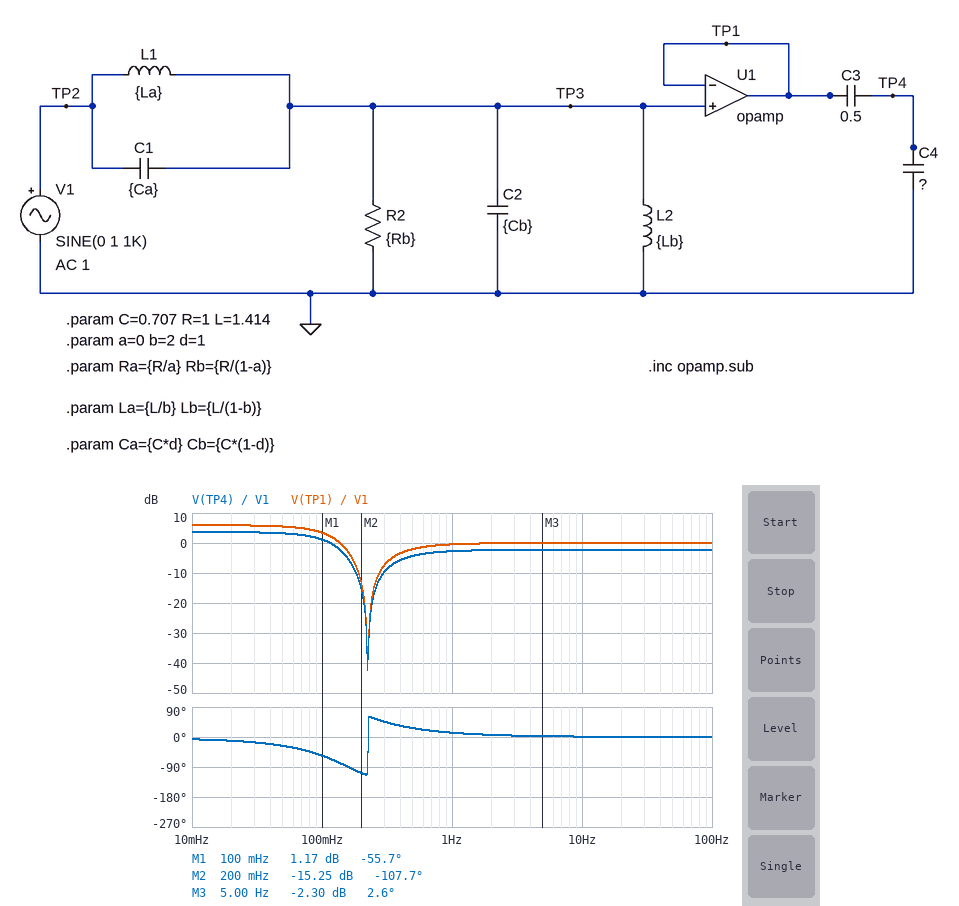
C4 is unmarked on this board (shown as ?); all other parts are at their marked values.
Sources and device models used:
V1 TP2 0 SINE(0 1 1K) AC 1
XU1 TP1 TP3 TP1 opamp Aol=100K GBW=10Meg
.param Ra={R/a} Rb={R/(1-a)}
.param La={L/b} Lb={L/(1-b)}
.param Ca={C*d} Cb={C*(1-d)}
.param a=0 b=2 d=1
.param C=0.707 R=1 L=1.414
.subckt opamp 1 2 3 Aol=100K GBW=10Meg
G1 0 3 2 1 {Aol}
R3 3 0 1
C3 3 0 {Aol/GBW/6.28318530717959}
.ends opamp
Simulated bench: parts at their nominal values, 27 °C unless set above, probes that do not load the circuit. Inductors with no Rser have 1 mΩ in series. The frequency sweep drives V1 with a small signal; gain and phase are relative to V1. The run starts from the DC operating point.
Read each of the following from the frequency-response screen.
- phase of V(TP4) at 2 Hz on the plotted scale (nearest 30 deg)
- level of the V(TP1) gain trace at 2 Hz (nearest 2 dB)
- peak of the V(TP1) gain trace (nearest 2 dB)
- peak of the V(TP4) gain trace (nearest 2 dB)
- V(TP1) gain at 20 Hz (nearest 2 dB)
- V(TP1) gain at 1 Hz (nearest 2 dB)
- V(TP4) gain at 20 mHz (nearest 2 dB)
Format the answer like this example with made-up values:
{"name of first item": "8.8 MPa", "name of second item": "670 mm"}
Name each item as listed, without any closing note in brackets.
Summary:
{"phase of V(TP4) at 2 Hz on the plotted scale": "0 deg", "level of the V(TP1) gain trace at 2 Hz": "0 dB", "peak of the V(TP1) gain trace": "6 dB", "peak of the V(TP4) gain trace": "4 dB", "V(TP1) gain at 20 Hz": "0 dB", "V(TP1) gain at 1 Hz": "0 dB", "V(TP4) gain at 20 mHz": "4 dB"}
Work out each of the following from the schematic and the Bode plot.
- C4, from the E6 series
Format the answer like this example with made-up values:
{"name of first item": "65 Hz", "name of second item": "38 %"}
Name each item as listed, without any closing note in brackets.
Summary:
{"C4, from the E6 series": "150 mF"}
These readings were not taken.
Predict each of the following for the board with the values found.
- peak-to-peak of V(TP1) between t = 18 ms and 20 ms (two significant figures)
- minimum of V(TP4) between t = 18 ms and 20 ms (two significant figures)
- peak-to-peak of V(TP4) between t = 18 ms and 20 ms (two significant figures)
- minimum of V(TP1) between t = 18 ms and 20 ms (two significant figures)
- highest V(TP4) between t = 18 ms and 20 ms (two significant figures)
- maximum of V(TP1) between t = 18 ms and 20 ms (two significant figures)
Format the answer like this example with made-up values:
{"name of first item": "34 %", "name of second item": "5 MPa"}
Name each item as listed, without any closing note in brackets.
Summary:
{"peak-to-peak of V(TP1) between t = 18 ms and 20 ms": "2.0 V", "minimum of V(TP4) between t = 18 ms and 20 ms": "-770 mV", "peak-to-peak of V(TP4) between t = 18 ms and 20 ms": "1.5 V", "minimum of V(TP1) between t = 18 ms and 20 ms": "-1.0 V", "highest V(TP4) between t = 18 ms and 20 ms": "770 mV", "maximum of V(TP1) between t = 18 ms and 20 ms": "1.0 V"}
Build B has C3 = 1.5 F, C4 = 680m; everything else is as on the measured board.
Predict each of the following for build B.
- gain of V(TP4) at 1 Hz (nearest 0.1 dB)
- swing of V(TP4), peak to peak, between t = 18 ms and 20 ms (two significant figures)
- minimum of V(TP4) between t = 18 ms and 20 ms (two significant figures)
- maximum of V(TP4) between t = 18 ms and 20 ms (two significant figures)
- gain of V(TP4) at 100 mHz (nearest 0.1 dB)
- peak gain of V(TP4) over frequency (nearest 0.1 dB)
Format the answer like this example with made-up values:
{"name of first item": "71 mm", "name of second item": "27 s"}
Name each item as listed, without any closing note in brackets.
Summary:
{"gain of V(TP4) at 1 Hz": "-3.7 dB", "swing of V(TP4), peak to peak, between t = 18 ms and 20 ms": "1.4 V", "minimum of V(TP4) between t = 18 ms and 20 ms": "-690 mV", "maximum of V(TP4) between t = 18 ms and 20 ms": "690 mV", "gain of V(TP4) at 100 mHz": "0.2 dB", "peak gain of V(TP4) over frequency": "2.7 dB"}
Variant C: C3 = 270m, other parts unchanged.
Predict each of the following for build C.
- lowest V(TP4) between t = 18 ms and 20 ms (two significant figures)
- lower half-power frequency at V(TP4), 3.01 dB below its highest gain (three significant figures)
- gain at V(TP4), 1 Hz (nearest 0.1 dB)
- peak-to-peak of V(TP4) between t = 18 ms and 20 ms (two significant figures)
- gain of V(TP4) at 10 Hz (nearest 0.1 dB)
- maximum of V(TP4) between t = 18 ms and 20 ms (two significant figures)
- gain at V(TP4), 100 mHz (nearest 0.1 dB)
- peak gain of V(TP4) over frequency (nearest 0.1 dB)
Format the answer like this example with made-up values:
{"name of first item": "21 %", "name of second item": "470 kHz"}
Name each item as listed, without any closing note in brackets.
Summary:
{"lowest V(TP4) between t = 18 ms and 20 ms": "-640 mV", "lower half-power frequency at V(TP4), 3.01 dB below its highest gain": "417 µHz", "gain at V(TP4), 1 Hz": "-4.3 dB", "peak-to-peak of V(TP4) between t = 18 ms and 20 ms": "1.3 V", "gain of V(TP4) at 10 Hz": "-3.8 dB", "maximum of V(TP4) between t = 18 ms and 20 ms": "640 mV", "gain at V(TP4), 100 mHz": "-0.4 dB", "peak gain of V(TP4) over frequency": "2.1 dB"}
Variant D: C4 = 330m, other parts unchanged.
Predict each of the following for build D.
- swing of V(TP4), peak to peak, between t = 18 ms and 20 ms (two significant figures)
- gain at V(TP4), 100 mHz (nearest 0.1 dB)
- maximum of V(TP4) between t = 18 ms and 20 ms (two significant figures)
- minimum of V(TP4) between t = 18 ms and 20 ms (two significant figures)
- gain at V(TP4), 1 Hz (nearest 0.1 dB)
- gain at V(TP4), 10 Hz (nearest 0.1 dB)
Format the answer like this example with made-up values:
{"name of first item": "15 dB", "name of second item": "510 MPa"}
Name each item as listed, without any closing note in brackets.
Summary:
{"swing of V(TP4), peak to peak, between t = 18 ms and 20 ms": "1.2 V", "gain at V(TP4), 100 mHz": "-1.0 dB", "maximum of V(TP4) between t = 18 ms and 20 ms": "600 mV", "minimum of V(TP4) between t = 18 ms and 20 ms": "-600 mV", "gain at V(TP4), 1 Hz": "-4.9 dB", "gain at V(TP4), 10 Hz": "-4.4 dB"}
